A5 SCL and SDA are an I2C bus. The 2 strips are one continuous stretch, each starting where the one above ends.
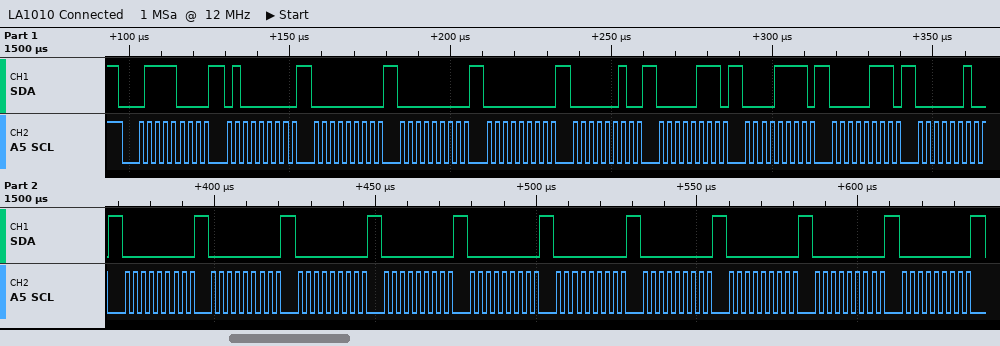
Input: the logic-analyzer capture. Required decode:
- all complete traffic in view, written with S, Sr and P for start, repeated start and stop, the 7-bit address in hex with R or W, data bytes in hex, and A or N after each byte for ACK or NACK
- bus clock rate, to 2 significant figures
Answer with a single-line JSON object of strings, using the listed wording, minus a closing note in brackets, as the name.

{"all complete traffic in view, written with S, Sr and P for start, repeated start and stop, the 7-bit address in hex with R or W, data bytes in hex, and A or N after each byte for ACK or NACK": "S 3CW A 40 A 00 A 00 A 00 A 02 A 07 A 0F A 07 A 02 A 00 A 00 A 00 A 00 A 00 A 00 A 00 A 00 A 00 A 00 A", "bus clock rate, to 2 significant figures": "400 kHz"}
